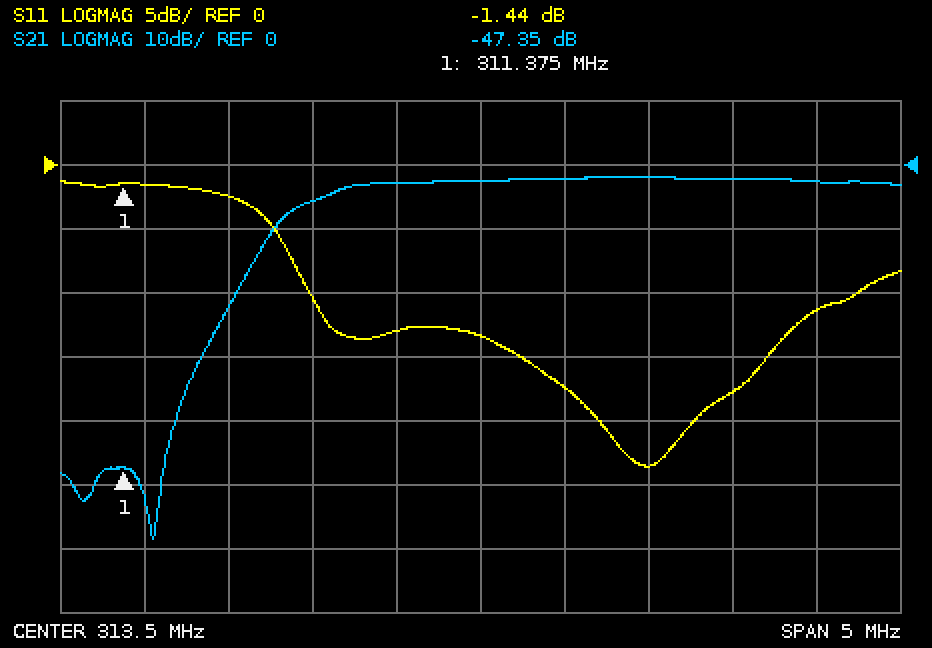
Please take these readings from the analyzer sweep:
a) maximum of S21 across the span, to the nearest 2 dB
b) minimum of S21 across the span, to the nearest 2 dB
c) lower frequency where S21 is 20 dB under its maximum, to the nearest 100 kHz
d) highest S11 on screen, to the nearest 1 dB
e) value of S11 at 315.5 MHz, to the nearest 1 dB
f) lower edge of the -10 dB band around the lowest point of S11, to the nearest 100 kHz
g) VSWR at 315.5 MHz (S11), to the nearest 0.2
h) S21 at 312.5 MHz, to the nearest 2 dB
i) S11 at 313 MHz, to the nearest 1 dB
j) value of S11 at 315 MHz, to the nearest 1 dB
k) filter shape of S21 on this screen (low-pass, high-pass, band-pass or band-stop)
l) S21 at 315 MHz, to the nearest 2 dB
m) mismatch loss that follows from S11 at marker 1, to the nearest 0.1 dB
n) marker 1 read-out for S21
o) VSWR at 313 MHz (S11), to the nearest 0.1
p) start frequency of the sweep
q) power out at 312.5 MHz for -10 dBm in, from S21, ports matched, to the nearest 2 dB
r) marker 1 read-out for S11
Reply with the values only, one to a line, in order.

-2 dB
-58 dB
312.0 MHz
-1 dB
-11 dB
312.5 MHz
1.8
-6 dB
-13 dB
-18 dB
high-pass
-2 dB
5.5 dB
-47.35 dB
1.6
311 MHz
-16 dBm
-1.44 dB
